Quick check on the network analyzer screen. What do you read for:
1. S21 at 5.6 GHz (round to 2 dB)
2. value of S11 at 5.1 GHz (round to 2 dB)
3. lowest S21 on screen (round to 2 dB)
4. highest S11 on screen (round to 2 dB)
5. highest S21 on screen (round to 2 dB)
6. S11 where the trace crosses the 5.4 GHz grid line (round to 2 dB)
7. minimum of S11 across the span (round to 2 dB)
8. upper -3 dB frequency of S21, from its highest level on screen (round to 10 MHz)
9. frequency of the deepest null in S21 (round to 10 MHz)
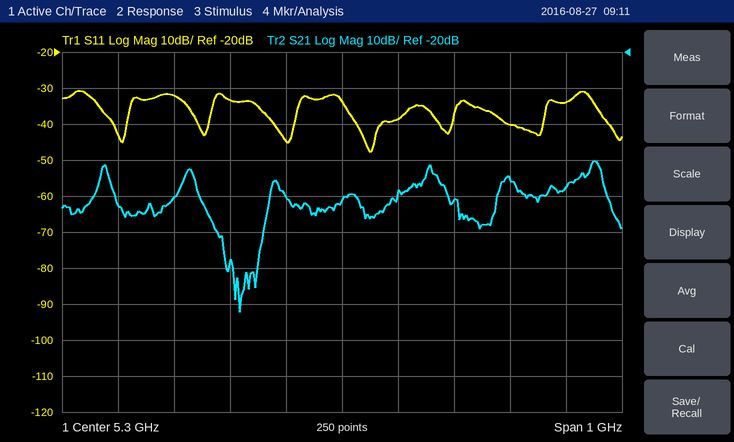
-56 dB
-34 dB
-92 dB
-30 dB
-50 dB
-38 dB
-48 dB
5.76 GHz
5.12 GHz
